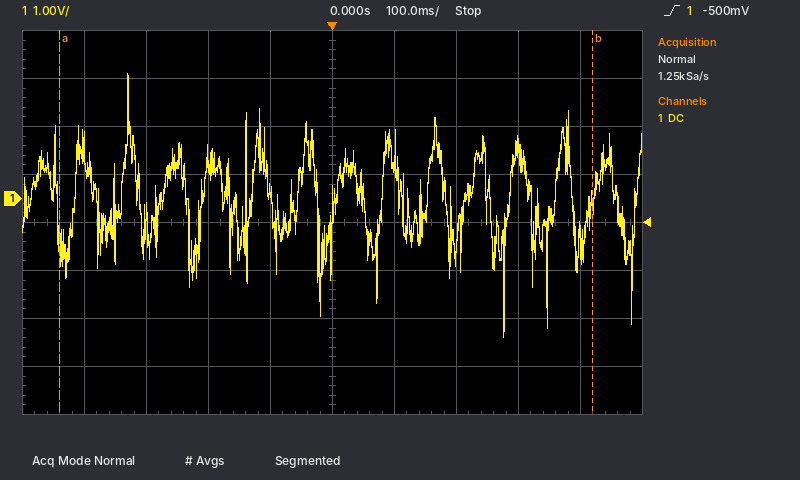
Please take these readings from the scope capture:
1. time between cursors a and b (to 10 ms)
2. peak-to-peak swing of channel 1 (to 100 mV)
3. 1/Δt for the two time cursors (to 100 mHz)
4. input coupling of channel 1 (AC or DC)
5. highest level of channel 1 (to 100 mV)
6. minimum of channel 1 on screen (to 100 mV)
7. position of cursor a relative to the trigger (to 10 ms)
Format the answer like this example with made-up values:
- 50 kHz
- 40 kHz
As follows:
- 860 ms
- 5.5 V
- 1.2 Hz
- DC
- 2.6 V
- -2.9 V
- -440 ms
